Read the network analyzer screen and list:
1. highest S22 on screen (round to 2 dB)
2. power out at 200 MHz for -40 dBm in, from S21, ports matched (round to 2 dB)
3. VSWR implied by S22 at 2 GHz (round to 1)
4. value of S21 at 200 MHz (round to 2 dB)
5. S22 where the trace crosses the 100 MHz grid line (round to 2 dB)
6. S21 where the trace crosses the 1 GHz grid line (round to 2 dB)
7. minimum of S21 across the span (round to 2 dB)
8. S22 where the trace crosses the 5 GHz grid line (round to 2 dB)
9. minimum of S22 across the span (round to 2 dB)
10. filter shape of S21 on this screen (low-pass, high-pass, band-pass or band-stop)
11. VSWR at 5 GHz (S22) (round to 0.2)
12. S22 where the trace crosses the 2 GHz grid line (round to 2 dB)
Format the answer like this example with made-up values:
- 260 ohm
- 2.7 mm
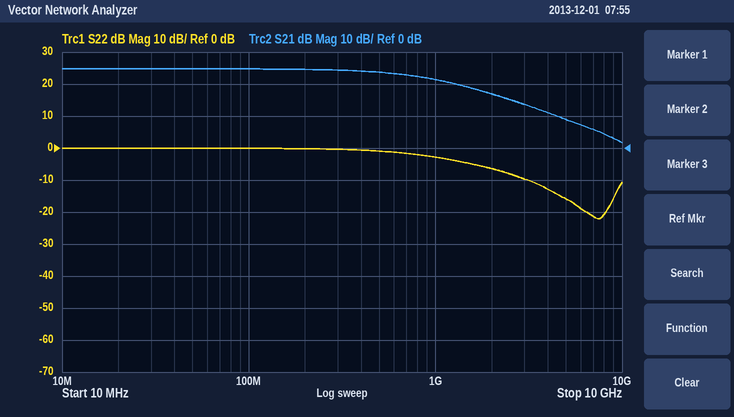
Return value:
- 0 dB
- -16 dBm
- 3
- 24 dB
- 0 dB
- 22 dB
- 2 dB
- -16 dB
- -22 dB
- low-pass
- 1.4
- -6 dB
